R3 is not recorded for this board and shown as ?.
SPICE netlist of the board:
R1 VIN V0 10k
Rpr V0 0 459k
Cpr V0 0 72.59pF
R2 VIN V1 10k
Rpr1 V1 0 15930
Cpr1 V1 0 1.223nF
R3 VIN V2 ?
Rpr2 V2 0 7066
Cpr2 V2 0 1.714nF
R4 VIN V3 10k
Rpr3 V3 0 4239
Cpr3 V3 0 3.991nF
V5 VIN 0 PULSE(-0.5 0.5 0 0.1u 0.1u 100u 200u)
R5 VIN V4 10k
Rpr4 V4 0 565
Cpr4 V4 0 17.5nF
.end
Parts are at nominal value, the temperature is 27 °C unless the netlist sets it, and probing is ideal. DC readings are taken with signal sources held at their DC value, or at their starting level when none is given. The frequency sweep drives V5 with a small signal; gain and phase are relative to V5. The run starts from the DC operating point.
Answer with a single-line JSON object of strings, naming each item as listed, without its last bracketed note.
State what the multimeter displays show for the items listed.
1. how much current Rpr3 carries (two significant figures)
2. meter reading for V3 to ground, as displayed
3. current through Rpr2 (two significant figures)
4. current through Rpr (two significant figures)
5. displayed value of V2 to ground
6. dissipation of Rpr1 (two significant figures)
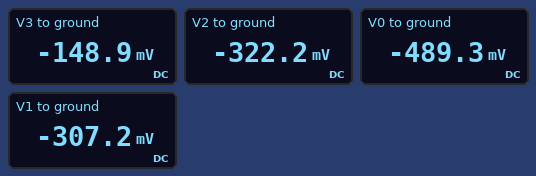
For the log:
{"how much current Rpr3 carries": "35 µA", "meter reading for V3 to ground, as displayed": "-148.9 mV", "current through Rpr2": "46 µA", "current through Rpr": "1.1 µA", "displayed value of V2 to ground": "-322.2 mV", "dissipation of Rpr1": "5.9 µW"}
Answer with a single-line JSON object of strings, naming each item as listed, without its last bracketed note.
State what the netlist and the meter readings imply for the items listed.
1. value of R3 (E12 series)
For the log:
{"value of R3": "3.9 kΩ"}
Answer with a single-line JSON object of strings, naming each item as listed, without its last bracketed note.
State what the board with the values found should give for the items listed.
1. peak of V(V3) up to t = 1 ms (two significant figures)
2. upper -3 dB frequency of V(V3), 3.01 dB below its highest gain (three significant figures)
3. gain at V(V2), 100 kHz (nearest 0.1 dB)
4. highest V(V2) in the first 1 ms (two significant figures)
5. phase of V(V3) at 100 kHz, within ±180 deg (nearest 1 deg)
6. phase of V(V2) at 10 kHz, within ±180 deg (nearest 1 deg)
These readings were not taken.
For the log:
{"peak of V(V3) up to t = 1 ms": "150 mV", "upper -3 dB frequency of V(V3), 3.01 dB below its highest gain": "13.4 kHz", "gain at V(V2), 100 kHz": "-13.0 dB", "highest V(V2) in the first 1 ms": "320 mV", "phase of V(V3) at 100 kHz, within ±180 deg": "-82 deg", "phase of V(V2) at 10 kHz, within ±180 deg": "-15 deg"}
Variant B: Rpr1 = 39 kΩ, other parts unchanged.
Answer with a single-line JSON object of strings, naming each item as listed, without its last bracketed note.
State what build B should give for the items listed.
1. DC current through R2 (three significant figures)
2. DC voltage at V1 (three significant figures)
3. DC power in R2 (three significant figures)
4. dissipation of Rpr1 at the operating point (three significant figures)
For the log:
{"DC current through R2": "10.2 µA", "DC voltage at V1": "-398 mV", "DC power in R2": "1.04 µW", "dissipation of Rpr1 at the operating point": "4.06 µW"}
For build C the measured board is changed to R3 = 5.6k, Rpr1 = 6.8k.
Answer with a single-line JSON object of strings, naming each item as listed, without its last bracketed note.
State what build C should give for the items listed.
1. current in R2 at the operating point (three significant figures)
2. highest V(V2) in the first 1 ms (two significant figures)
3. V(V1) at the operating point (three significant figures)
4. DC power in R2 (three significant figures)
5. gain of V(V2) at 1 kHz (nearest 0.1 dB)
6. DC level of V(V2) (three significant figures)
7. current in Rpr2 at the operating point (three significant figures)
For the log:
{"current in R2 at the operating point": "29.8 µA", "highest V(V2) in the first 1 ms": "280 mV", "V(V1) at the operating point": "-202 mV", "DC power in R2": "8.86 µW", "gain of V(V2) at 1 kHz": "-5.1 dB", "DC level of V(V2)": "-279 mV", "current in Rpr2 at the operating point": "39.5 µA"}
